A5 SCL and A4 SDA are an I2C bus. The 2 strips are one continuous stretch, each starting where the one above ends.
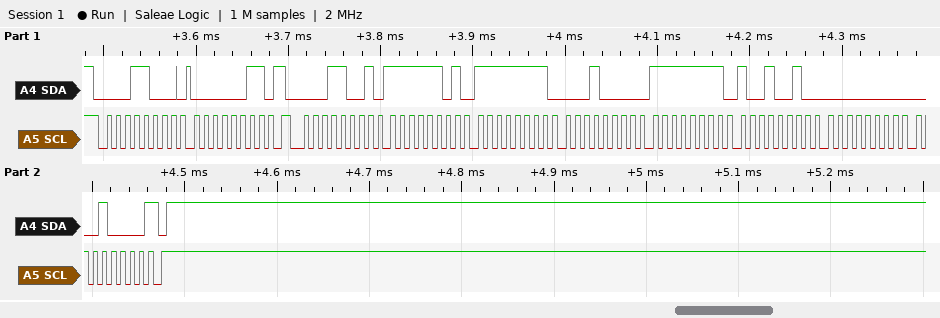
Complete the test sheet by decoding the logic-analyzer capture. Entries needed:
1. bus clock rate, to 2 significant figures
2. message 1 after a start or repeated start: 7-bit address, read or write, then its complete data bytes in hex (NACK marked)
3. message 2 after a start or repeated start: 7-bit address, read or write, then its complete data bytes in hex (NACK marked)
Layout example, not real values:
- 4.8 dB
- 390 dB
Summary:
- 100 kHz
- 0x0C write: 03
- 0x0C read: FD FF 10 FF 92 00 10 NACK
